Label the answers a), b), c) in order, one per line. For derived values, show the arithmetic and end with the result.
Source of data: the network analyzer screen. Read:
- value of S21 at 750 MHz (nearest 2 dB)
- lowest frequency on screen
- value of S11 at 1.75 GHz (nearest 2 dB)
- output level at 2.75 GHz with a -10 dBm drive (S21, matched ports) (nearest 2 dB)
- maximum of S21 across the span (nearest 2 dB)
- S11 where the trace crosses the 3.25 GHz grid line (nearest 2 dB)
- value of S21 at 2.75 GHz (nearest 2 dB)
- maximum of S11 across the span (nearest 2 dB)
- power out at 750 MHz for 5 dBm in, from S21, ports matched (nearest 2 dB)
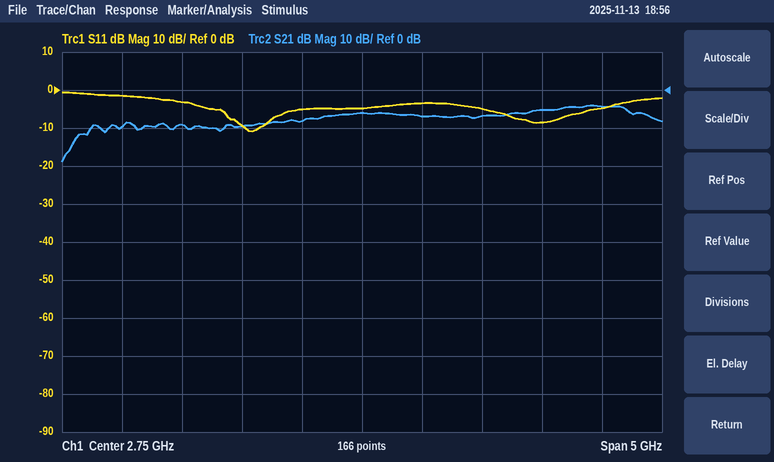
a) -10 dB
b) 250 MHz
c) -10 dB
d) -10 dBm + (-6 dB) = -16 dBm
e) -4 dB
f) -4 dB
g) -6 dB
h) 0 dB
i) 5 dBm + (-10 dB) = -4 dBm
